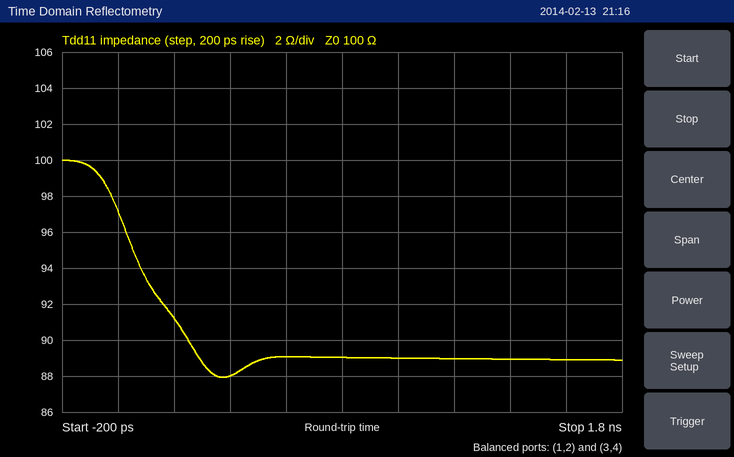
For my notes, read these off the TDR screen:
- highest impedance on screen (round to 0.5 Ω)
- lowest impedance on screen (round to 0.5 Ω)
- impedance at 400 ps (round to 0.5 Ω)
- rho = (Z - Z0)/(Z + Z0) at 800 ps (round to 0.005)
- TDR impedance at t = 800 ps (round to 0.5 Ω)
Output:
100.0 Ω
88.0 Ω
88.0 Ω
-0.060
89.0 Ω
